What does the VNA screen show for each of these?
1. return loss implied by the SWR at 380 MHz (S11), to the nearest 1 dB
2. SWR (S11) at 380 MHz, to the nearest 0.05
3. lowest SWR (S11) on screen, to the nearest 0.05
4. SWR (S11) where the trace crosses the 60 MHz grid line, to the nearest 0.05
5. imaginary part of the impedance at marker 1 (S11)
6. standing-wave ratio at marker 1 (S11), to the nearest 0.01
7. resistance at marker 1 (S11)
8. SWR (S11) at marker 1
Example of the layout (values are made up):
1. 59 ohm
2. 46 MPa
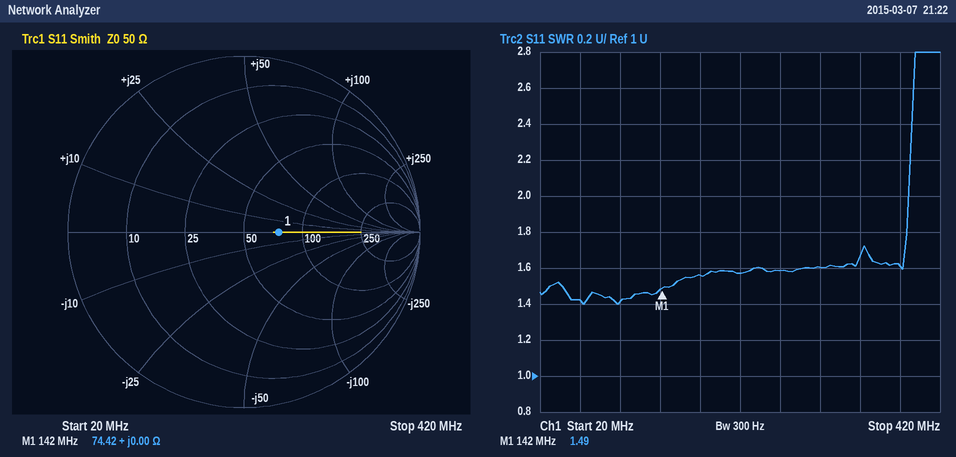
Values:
1. 13 dB
2. 1.60
3. 1.40
4. 1.40
5. +0.00 Ω
6. 1.49
7. 74.42 Ω
8. 1.49
